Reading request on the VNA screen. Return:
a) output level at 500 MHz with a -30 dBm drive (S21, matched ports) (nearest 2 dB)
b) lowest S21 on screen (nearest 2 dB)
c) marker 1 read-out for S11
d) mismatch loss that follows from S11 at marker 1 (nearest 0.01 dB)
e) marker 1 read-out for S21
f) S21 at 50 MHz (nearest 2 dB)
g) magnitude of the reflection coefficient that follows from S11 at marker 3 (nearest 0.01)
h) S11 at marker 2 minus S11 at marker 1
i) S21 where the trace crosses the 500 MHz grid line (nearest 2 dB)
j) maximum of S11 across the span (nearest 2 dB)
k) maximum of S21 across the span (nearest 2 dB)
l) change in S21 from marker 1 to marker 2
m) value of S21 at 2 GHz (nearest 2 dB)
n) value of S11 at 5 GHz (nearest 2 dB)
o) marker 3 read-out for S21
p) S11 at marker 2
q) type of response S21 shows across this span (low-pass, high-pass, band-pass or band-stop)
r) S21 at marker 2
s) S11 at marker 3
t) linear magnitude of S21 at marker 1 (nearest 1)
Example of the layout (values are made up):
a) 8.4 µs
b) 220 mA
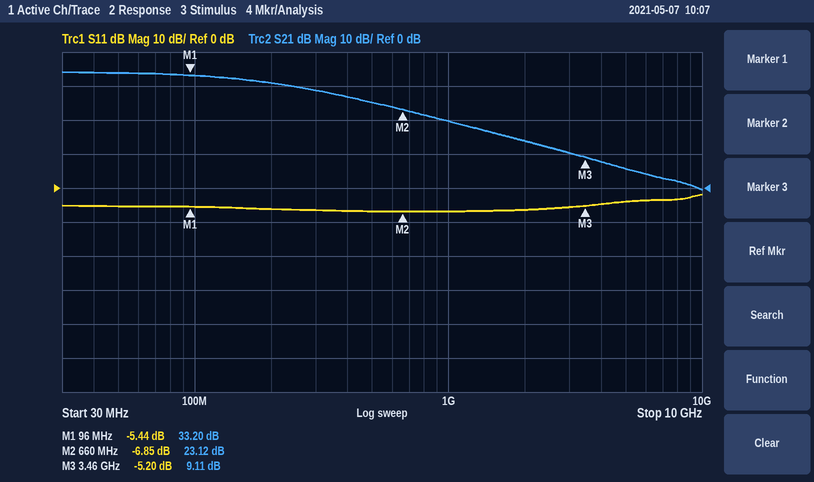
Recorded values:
a) -4 dBm
b) 0 dB
c) -5.44 dB
d) 1.46 dB
e) 33.20 dB
f) 34 dB
g) 0.55
h) -1.41 dB
i) 26 dB
j) -2 dB
k) 34 dB
l) -10.08 dB
m) 14 dB
n) -4 dB
o) 9.11 dB
p) -6.85 dB
q) low-pass
r) 23.12 dB
s) -5.20 dB
t) 46
